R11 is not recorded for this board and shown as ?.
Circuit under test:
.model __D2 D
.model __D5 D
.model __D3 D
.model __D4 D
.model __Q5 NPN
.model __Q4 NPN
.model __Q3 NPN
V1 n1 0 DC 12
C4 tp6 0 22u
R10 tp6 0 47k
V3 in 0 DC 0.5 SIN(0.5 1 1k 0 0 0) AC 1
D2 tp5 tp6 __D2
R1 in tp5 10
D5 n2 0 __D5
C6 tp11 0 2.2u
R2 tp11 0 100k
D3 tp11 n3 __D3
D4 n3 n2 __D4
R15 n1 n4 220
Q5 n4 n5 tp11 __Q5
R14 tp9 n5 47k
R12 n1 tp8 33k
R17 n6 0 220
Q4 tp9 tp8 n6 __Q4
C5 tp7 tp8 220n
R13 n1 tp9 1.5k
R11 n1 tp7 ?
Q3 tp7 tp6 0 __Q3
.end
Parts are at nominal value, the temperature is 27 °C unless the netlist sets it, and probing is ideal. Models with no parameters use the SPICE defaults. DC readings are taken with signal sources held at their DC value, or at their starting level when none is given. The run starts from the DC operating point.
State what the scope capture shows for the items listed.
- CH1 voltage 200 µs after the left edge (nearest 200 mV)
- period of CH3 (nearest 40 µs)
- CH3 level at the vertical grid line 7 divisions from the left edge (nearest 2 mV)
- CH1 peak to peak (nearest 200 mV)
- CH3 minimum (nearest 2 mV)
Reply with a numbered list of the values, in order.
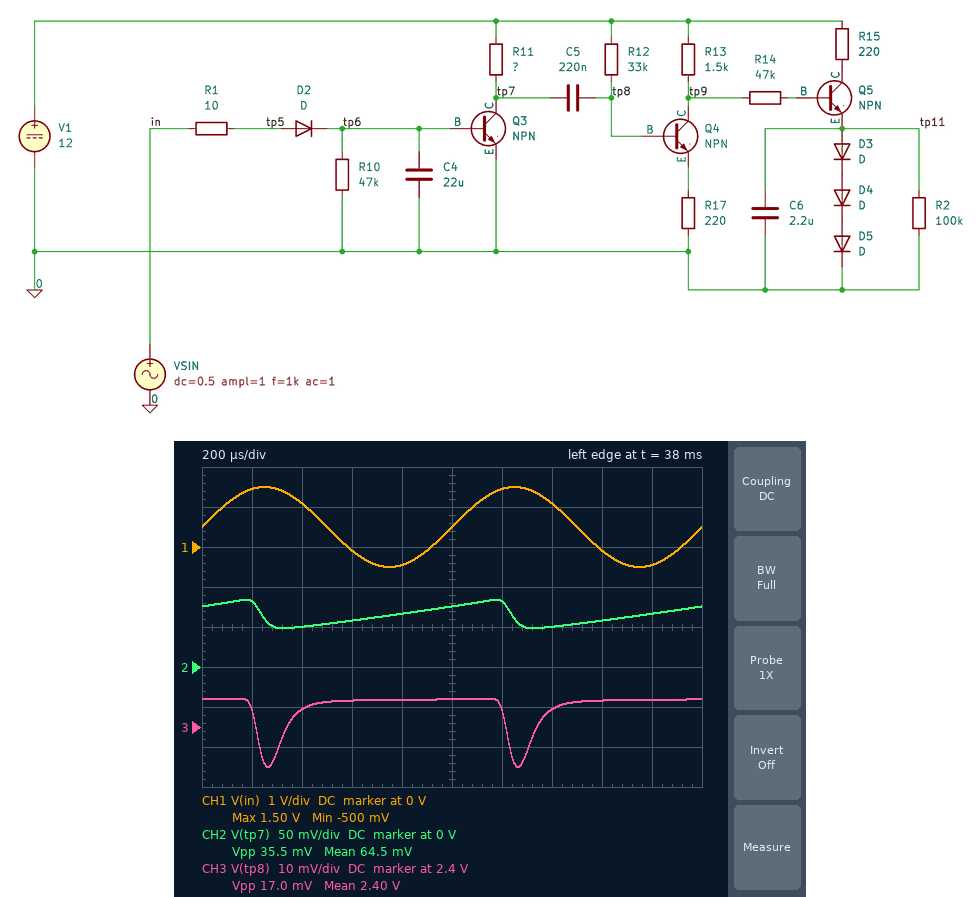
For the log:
1. 1.4 V
2. 1.00 ms
3. 2.404 V
4. 2.0 V
5. 2.390 V
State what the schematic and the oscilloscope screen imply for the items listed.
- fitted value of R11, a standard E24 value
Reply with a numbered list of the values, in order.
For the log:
1. 7.5 kΩ
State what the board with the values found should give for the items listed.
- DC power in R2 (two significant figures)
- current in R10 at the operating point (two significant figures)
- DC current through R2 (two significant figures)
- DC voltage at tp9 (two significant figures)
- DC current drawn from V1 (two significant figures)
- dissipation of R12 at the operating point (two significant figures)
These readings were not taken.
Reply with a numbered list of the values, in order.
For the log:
1. 10 µW
2. 700 nA
3. 10 µA
4. 1.7 V
5. 7.2 mA
6. 2.8 mW
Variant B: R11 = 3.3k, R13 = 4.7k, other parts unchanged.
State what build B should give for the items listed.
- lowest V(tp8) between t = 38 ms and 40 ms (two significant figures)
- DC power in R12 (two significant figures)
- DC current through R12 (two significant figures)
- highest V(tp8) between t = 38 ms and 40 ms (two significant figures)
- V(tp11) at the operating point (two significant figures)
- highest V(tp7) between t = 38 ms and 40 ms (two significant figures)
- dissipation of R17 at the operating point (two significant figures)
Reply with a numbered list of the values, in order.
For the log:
1. 1.3 V
2. 3.4 mW
3. 320 µA
4. 1.4 V
5. 74 mV
6. 220 mV
7. 1.6 mW
